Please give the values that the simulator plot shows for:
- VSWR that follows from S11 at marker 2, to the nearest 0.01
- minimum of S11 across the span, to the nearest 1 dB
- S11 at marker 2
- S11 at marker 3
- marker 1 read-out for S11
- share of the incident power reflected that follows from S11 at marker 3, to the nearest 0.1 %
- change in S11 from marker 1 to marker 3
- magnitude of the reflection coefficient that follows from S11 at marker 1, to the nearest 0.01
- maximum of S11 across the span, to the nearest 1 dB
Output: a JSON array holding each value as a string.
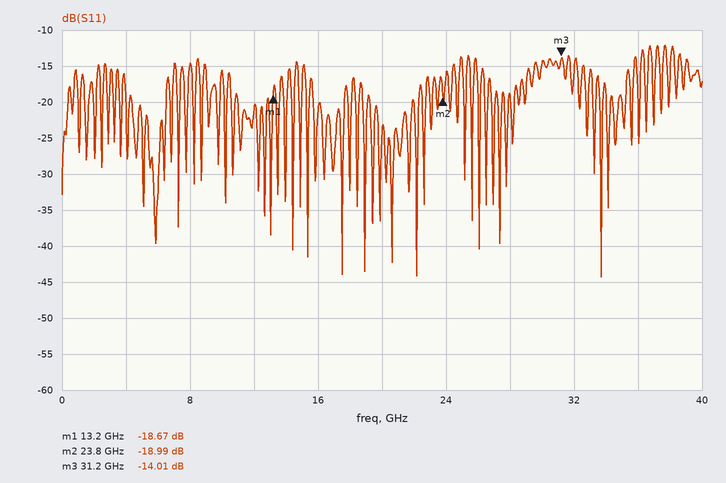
["1.25", "-44 dB", "-18.99 dB", "-14.01 dB", "-18.67 dB", "4.0 %", "4.66 dB", "0.12", "-12 dB"]
